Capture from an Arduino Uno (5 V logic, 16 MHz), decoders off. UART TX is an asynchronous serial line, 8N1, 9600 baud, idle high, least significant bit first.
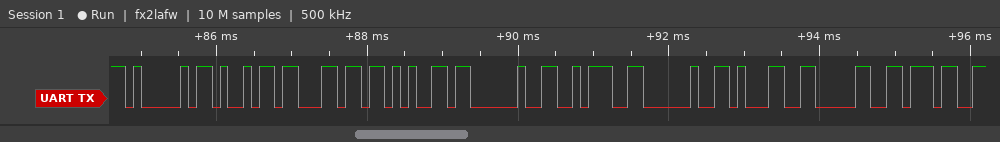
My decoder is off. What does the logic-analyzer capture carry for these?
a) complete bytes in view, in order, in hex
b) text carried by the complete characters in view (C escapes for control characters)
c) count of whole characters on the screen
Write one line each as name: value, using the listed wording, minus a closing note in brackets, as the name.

complete bytes in view, in order, in hex: 0x41 0x69 0x6C 0x65 0x20 0x3A 0x20 0x31 0x30 0x37
text carried by the complete characters in view: "Aile : 107"
count of whole characters on the screen: 10
